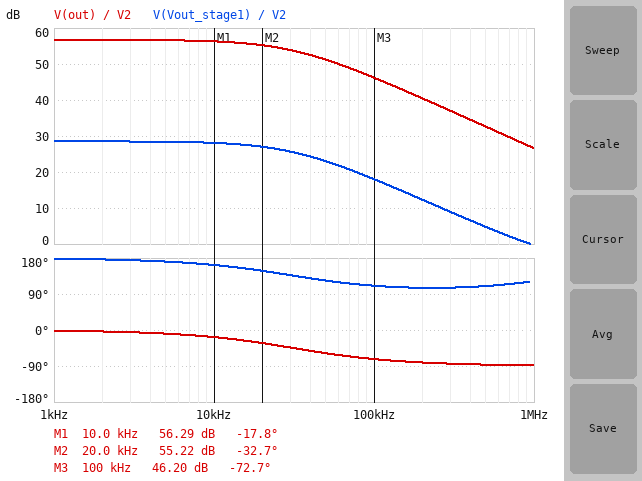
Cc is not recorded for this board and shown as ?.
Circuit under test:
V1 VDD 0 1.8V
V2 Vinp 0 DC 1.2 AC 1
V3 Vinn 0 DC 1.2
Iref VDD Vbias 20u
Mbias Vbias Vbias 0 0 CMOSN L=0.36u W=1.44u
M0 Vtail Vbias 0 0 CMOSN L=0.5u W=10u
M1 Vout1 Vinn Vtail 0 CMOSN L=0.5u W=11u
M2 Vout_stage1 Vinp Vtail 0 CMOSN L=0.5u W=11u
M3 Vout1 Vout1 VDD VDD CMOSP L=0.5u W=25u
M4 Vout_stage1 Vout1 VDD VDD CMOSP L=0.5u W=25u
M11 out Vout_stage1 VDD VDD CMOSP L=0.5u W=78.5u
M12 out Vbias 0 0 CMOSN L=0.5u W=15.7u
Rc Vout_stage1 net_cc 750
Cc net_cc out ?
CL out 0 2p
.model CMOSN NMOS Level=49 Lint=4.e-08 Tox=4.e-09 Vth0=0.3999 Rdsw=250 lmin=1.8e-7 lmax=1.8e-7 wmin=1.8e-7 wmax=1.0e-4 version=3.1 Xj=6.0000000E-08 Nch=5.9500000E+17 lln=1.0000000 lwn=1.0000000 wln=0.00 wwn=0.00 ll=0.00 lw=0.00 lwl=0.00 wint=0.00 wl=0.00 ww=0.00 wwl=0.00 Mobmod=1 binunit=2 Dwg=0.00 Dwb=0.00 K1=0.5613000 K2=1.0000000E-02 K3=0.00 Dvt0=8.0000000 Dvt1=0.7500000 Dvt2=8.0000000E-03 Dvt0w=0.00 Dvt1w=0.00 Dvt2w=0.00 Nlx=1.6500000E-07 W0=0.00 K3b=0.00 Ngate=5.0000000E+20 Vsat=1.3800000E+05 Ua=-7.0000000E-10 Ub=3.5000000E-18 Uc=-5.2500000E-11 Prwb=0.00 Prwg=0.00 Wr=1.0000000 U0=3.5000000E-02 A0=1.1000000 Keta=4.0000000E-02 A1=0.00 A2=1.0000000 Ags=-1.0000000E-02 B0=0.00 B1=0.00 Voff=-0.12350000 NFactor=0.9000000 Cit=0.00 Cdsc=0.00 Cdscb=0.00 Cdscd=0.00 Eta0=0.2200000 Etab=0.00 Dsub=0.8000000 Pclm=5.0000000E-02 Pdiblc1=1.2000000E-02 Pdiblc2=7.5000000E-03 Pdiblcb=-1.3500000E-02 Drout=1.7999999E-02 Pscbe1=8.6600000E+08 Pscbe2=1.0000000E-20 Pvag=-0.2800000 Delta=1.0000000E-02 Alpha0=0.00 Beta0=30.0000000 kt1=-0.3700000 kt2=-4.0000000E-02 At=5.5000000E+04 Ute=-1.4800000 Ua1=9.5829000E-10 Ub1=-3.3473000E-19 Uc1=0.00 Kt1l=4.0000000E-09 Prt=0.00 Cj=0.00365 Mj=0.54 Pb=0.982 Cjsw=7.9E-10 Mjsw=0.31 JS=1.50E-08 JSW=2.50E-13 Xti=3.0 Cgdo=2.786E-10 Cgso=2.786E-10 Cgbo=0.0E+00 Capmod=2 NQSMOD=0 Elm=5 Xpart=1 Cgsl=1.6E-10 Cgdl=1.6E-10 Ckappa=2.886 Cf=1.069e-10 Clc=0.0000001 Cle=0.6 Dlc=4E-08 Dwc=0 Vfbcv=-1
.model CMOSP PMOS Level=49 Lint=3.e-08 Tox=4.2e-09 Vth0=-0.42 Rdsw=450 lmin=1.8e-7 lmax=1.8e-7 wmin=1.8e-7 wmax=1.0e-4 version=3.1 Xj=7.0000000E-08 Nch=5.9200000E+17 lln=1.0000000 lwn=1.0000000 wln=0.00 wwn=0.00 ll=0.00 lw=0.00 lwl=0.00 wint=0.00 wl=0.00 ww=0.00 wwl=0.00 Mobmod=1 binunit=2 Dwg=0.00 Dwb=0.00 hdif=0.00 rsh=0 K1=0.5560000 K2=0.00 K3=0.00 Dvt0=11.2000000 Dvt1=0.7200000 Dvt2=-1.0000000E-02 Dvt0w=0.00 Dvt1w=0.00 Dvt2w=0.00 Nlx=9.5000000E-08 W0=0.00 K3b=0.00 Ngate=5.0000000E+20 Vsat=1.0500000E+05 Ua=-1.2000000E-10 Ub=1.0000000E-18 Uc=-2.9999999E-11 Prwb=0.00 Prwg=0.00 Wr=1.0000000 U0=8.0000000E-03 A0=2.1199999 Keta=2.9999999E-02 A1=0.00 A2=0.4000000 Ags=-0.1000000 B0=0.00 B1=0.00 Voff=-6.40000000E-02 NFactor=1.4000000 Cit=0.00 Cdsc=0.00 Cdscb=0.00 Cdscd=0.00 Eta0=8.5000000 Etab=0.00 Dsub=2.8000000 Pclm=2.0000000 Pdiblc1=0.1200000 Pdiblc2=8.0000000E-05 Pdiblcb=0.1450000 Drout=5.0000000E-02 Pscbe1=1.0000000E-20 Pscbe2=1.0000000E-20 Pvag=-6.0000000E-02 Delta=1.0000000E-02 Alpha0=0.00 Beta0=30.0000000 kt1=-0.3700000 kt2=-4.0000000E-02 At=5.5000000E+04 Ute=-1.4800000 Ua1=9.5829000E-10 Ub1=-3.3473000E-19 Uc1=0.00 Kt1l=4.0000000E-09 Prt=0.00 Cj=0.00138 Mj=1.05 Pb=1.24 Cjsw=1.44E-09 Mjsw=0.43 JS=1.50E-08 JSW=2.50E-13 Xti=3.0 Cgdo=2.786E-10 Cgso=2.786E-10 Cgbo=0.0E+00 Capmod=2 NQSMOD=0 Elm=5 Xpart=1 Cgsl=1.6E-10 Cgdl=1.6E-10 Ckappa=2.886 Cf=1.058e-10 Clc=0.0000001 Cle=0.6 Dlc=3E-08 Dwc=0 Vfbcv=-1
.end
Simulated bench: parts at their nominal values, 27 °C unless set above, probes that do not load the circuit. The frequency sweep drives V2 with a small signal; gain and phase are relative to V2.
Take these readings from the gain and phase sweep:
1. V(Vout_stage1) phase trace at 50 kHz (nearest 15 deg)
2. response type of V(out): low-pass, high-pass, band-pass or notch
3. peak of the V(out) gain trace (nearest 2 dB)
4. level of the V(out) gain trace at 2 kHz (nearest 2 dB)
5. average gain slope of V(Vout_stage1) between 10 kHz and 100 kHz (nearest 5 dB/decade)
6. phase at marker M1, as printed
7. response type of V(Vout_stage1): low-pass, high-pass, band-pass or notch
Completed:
120 deg
low-pass
56 dB
56 dB
-10 dB/decade
-17.8 deg
low-pass
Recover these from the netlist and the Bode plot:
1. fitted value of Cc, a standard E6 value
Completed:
4.7 pF
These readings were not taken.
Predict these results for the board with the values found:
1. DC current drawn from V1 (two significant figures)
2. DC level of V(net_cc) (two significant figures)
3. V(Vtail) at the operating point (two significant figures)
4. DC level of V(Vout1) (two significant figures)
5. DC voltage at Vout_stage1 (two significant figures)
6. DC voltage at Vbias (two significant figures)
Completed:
340 µA
1.1 V
460 mV
1.1 V
1.1 V
690 mV
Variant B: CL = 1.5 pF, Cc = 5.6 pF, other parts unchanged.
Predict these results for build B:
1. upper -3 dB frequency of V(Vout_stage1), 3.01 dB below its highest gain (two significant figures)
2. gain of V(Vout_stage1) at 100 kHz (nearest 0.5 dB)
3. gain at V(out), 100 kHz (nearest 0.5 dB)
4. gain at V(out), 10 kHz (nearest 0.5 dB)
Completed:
26 kHz
16.5 dB
45.0 dB
56.0 dB
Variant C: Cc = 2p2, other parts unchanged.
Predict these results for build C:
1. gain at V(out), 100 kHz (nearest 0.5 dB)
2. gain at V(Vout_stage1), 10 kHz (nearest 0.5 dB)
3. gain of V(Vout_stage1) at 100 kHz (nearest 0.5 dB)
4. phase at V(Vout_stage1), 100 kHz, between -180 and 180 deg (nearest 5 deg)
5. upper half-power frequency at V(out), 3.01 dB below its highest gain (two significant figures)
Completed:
51.5 dB
28.5 dB
23.5 dB
125 deg
65 kHz
